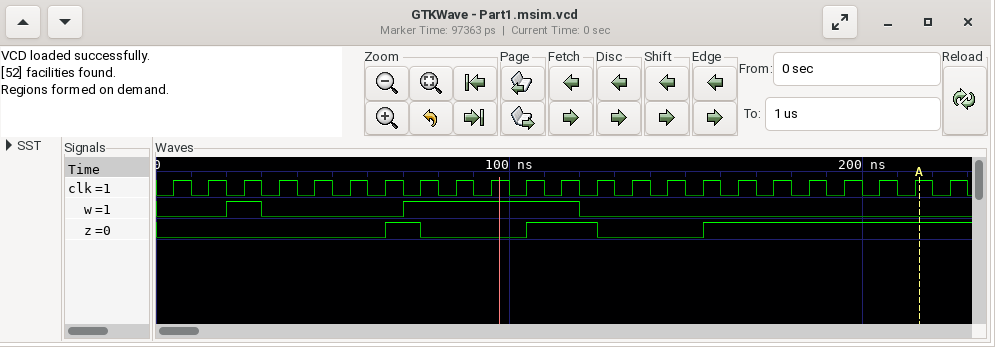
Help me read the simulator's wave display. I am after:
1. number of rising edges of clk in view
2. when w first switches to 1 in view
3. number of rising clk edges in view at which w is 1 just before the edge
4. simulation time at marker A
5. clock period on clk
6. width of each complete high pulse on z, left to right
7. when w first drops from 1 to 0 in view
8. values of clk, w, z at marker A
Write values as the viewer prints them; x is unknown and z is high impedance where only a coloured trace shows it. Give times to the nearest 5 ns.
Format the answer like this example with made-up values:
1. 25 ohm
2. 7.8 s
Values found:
1. 23
2. 20 ns
3. 6
4. 215 ns
5. 10 ns
6. 10 ns, 20 ns
7. 30 ns
8. clk=1, w=0, z=1
